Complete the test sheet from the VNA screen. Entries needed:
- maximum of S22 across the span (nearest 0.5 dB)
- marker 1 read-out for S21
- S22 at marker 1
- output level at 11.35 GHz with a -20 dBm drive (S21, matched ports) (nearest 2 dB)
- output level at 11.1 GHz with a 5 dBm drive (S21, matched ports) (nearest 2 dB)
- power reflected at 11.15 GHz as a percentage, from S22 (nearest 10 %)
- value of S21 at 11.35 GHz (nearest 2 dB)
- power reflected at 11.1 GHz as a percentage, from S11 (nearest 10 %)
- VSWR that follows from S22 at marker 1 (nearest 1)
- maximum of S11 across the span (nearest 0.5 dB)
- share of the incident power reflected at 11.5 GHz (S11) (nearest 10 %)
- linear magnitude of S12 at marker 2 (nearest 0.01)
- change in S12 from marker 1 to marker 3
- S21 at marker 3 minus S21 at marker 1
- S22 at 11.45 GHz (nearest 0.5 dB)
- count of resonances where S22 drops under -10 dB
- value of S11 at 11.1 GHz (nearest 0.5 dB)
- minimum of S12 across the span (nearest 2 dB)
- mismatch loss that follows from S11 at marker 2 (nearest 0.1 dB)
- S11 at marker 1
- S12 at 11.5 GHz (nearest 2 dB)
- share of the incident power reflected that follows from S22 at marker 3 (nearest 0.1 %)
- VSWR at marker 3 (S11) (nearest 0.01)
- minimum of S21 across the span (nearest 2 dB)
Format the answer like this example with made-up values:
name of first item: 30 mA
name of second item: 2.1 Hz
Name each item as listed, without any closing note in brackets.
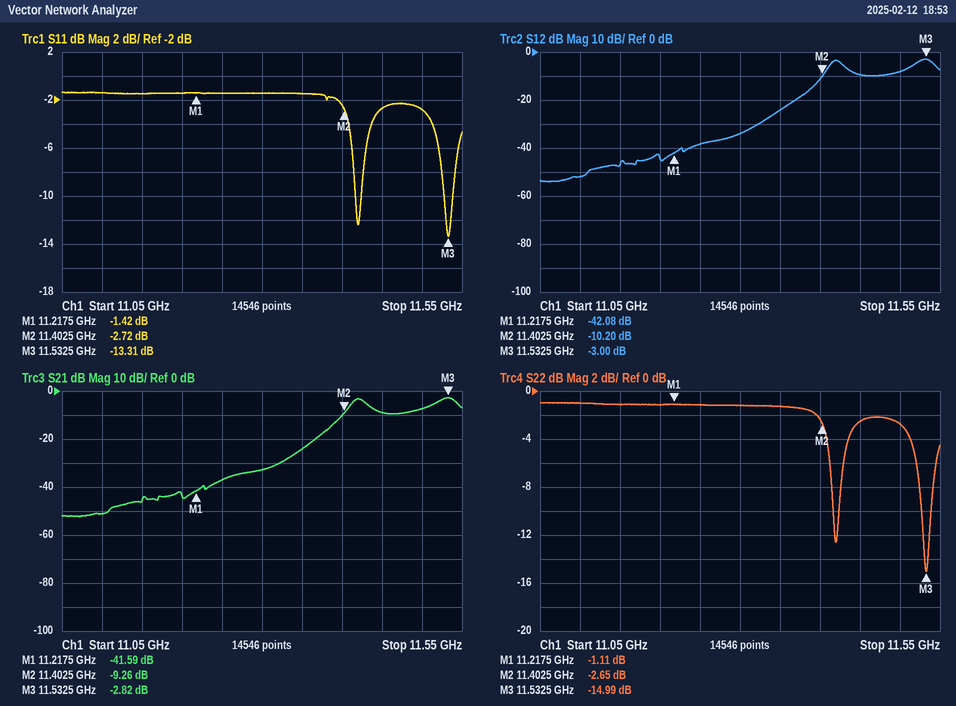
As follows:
maximum of S22 across the span: -1.0 dB
marker 1 read-out for S21: -41.59 dB
S22 at marker 1: -1.11 dB
output level at 11.35 GHz with a -20 dBm drive (S21, matched ports): -44 dBm
output level at 11.1 GHz with a 5 dBm drive (S21, matched ports): -46 dBm
power reflected at 11.15 GHz as a percentage, from S22: 80 %
value of S21 at 11.35 GHz: -24 dB
power reflected at 11.1 GHz as a percentage, from S11: 70 %
VSWR that follows from S22 at marker 1: 16
maximum of S11 across the span: -1.5 dB
share of the incident power reflected at 11.5 GHz (S11): 50 %
linear magnitude of S12 at marker 2: 0.31
change in S12 from marker 1 to marker 3: 39.08 dB
S21 at marker 3 minus S21 at marker 1: 38.77 dB
S22 at 11.45 GHz: -2.5 dB
count of resonances where S22 drops under -10 dB: 2
value of S11 at 11.1 GHz: -1.5 dB
minimum of S12 across the span: -54 dB
mismatch loss that follows from S11 at marker 2: 3.3 dB
S11 at marker 1: -1.42 dB
S12 at 11.5 GHz: -8 dB
share of the incident power reflected that follows from S22 at marker 3: 3.2 %
VSWR at marker 3 (S11): 1.55
minimum of S21 across the span: -52 dB
